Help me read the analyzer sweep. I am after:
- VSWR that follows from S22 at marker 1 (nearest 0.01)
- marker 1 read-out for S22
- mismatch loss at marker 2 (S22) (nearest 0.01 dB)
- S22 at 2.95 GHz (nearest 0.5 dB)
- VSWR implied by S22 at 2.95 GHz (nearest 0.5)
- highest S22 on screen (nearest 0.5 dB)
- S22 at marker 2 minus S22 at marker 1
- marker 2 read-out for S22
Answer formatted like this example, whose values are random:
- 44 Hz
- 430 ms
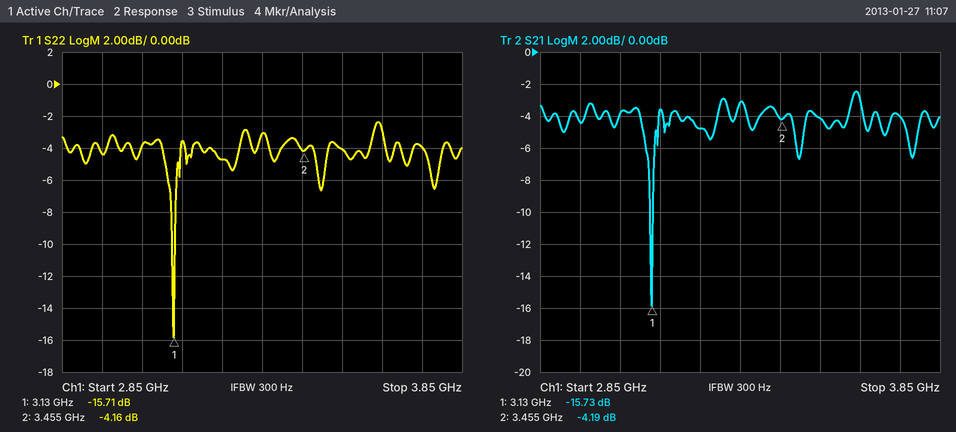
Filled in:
- 1.39
- -15.71 dB
- 2.10 dB
- -4.5 dB
- 4.0
- -2.5 dB
- 11.55 dB
- -4.16 dB
